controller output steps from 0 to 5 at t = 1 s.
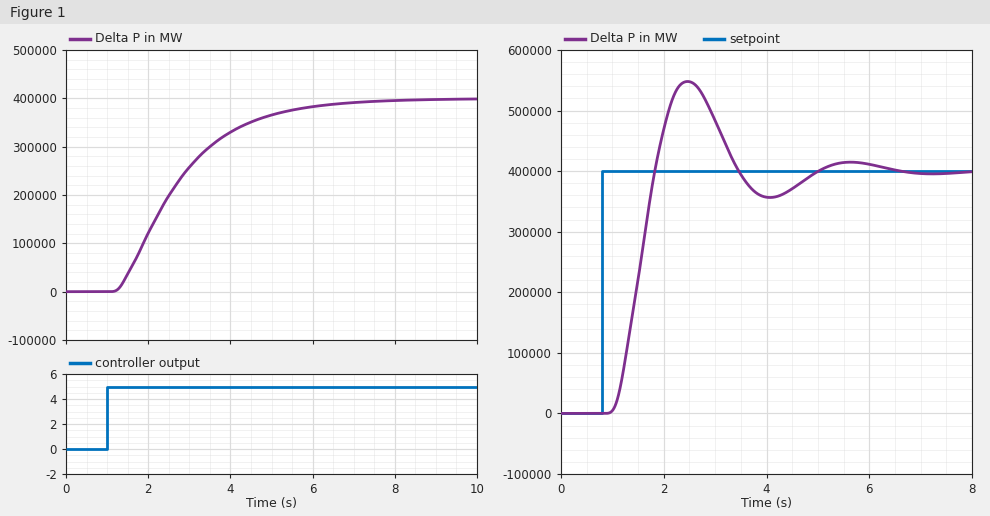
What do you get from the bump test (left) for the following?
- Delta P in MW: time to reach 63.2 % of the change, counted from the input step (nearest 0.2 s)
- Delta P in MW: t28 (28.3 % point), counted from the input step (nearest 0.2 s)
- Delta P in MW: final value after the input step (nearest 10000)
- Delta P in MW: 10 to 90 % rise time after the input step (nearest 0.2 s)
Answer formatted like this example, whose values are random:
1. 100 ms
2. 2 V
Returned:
1. 2.0 s
2. 1.0 s
3. 400000
4. 3.2 s
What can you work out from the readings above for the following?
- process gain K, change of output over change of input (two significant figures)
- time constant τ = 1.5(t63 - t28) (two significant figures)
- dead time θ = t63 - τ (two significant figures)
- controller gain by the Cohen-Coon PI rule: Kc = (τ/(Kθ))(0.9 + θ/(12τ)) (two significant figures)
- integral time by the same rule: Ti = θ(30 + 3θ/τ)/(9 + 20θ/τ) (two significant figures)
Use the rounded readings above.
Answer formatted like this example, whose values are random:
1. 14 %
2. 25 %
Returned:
1. 80000
2. 1.5 s
3. 0.50 s
4. 0.000035
5. 0.99 s
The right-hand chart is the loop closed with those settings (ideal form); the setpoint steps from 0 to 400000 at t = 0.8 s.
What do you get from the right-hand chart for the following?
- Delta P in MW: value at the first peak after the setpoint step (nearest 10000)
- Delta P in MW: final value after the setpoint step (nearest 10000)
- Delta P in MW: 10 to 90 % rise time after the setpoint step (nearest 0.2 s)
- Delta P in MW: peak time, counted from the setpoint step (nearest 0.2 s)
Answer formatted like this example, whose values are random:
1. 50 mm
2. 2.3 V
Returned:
1. 550000
2. 400000
3. 0.6 s
4. 1.6 s
